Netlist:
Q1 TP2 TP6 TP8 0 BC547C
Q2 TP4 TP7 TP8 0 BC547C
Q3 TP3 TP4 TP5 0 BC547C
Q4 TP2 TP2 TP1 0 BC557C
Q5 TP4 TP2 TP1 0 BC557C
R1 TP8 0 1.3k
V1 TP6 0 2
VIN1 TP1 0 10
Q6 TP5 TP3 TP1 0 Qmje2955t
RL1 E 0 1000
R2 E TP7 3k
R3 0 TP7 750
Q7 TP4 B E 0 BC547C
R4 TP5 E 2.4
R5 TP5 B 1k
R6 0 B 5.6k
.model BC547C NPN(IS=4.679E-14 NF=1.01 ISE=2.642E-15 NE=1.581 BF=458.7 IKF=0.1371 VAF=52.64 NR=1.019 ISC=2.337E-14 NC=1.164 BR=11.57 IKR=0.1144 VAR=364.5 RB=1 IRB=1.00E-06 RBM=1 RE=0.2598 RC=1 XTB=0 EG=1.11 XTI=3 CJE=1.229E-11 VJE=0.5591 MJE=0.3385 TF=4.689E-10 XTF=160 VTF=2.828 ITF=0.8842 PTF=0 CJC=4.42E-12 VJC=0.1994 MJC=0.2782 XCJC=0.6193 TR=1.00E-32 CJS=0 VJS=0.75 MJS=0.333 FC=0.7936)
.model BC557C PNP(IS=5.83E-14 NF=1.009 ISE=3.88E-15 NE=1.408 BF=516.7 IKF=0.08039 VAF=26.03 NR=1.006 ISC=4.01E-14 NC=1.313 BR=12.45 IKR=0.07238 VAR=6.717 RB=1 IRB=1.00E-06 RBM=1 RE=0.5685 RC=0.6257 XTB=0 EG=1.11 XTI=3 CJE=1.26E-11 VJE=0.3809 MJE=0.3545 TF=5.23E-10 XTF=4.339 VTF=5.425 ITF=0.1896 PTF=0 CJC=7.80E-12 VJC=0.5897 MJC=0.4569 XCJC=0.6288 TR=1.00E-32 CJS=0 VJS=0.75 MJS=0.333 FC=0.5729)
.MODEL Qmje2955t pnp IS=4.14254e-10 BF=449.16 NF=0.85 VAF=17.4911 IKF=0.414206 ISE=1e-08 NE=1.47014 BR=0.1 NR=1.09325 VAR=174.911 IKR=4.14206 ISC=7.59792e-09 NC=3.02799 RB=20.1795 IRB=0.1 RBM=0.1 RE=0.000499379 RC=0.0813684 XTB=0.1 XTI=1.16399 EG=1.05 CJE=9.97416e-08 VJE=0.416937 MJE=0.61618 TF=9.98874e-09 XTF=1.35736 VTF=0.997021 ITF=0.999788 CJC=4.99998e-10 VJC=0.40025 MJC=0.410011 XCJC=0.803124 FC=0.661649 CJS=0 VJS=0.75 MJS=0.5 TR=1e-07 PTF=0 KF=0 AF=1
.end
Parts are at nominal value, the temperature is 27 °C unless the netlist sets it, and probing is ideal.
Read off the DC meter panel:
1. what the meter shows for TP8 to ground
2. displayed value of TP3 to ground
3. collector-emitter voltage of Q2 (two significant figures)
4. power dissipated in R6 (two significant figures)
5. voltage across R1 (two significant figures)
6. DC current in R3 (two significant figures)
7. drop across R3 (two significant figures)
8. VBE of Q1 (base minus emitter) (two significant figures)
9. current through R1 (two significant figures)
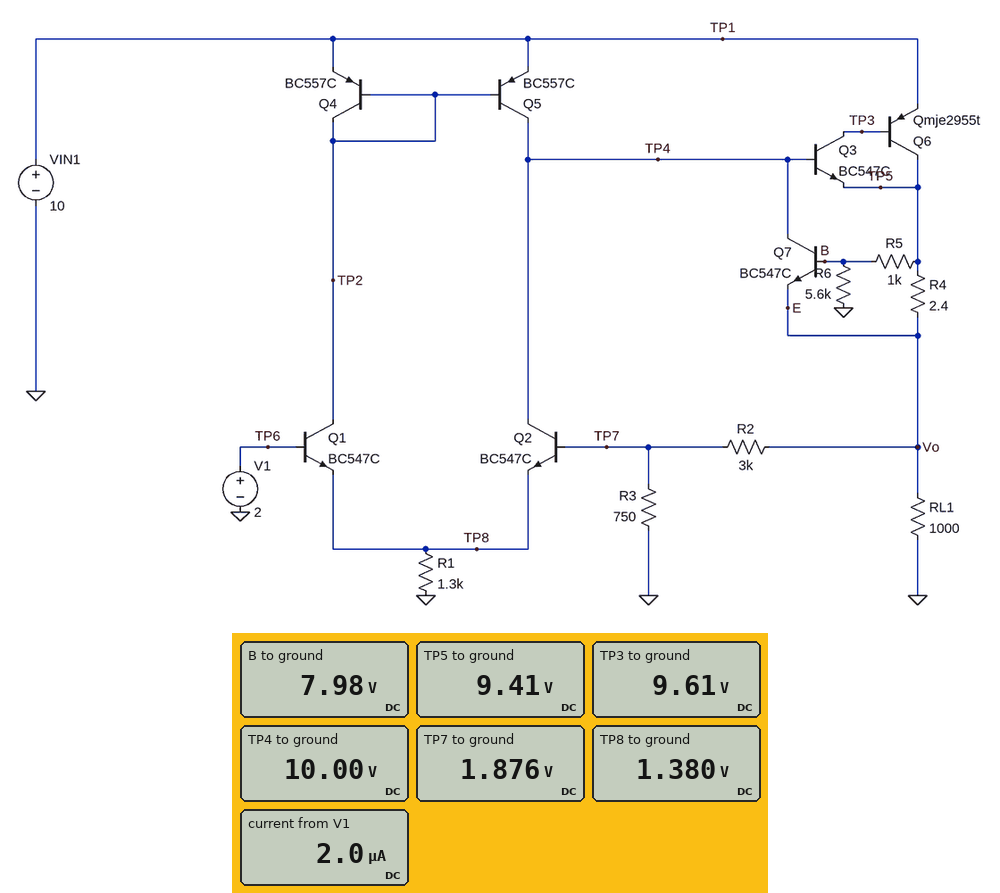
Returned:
1.380 V
9.61 V
8.6 V
11 mW
1.4 V
2.5 mA
1.9 V
620 mV
1.1 mA
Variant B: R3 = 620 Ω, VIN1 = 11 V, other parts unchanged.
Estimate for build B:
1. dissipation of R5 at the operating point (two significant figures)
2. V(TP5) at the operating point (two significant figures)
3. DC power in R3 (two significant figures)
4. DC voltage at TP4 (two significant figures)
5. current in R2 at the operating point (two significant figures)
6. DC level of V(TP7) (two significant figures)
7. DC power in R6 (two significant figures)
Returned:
2.5 mW
10 V
5.1 mW
11 V
2.9 mA
1.8 V
14 mW
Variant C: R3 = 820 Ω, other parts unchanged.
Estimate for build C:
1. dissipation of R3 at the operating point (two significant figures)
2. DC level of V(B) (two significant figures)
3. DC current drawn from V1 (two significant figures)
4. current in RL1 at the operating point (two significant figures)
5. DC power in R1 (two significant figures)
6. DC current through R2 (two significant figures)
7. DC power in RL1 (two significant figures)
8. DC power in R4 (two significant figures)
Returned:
4.9 mW
7.9 V
1.1 µA
9.3 mA
1.5 mW
2.4 mA
87 mW
330 µW
